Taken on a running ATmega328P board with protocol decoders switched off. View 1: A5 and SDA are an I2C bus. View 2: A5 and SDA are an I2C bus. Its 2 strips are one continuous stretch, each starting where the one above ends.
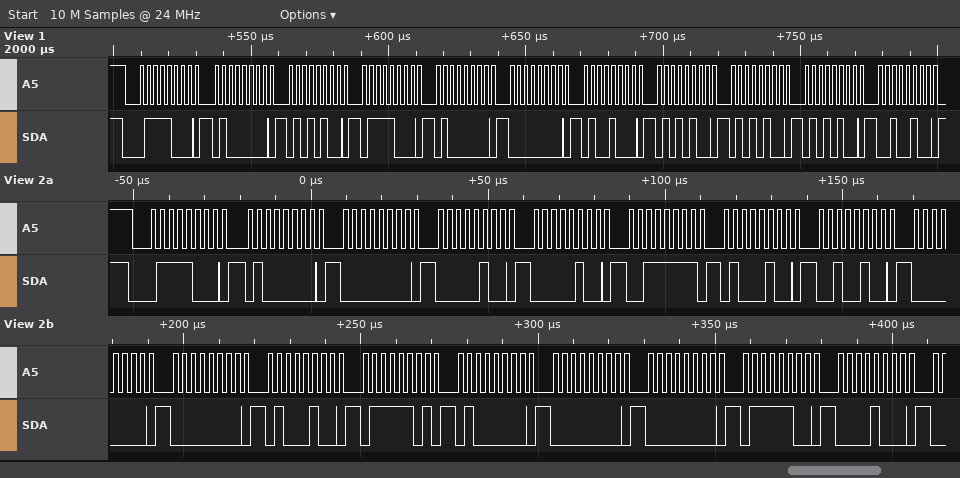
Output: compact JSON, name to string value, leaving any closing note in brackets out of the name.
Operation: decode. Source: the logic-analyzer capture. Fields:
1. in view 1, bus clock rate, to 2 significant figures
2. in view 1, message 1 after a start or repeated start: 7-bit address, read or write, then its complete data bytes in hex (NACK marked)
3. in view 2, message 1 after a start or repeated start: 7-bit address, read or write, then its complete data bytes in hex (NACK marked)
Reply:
{"in view 1, bus clock rate, to 2 significant figures": "400 kHz", "in view 1, message 1 after a start or repeated start: 7-bit address, read or write, then its complete data bytes in hex": "0x3C write: 40 54 78 40 00 48 54 54 54 24", "in view 2, message 1 after a start or repeated start: 7-bit address, read or write, then its complete data bytes in hex": "0x3C write: 40 00 04 04 3F 44 24 00 00 44 7D 40 00 00 7C 08"}
